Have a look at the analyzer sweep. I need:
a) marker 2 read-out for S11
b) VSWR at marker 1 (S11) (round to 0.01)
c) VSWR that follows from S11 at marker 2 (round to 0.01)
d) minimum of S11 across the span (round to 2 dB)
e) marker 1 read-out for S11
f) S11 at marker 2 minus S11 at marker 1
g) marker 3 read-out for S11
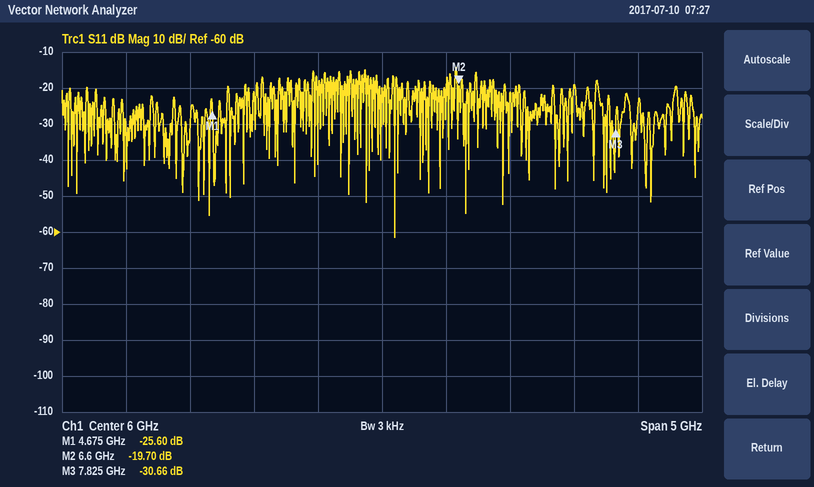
-19.70 dB
1.11
1.23
-62 dB
-25.60 dB
5.90 dB
-30.66 dB
